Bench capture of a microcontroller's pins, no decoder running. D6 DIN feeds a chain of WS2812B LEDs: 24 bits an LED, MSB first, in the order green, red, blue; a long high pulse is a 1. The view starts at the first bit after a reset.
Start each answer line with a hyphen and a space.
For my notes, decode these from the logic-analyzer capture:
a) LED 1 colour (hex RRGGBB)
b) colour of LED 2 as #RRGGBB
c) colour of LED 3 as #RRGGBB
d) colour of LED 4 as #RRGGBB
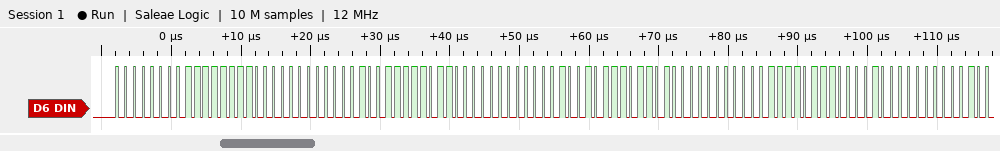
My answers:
- #FF0000
- #F60900
- #ED1200
- #E11E00
